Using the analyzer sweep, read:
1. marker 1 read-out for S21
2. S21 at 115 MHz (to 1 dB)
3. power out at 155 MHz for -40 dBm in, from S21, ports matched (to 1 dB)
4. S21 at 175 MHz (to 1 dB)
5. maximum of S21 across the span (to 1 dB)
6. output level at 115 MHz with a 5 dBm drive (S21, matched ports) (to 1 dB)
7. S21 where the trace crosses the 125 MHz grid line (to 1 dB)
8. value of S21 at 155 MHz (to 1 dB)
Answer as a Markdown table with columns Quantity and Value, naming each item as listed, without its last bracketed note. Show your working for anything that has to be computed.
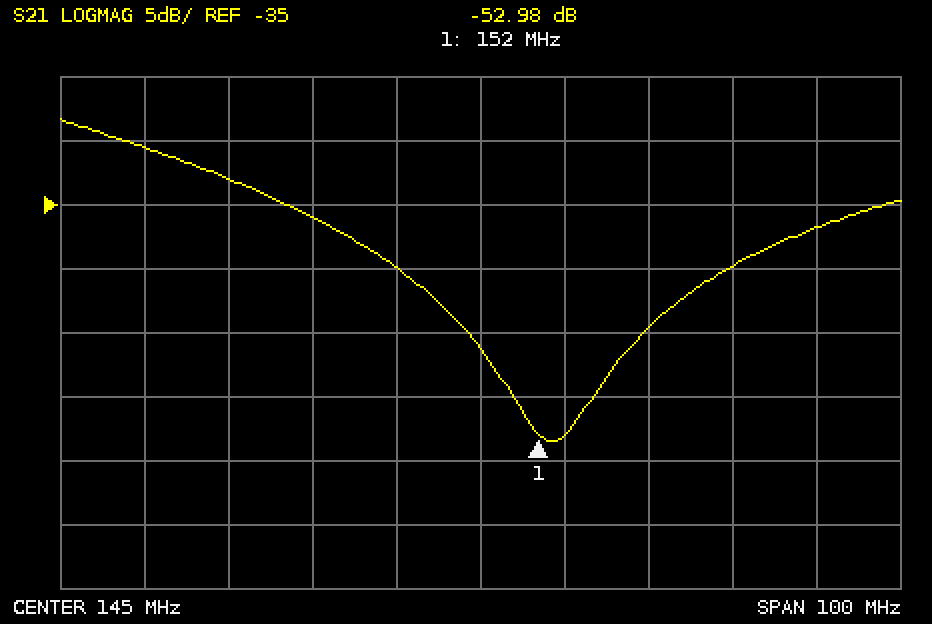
| Quantity | Value |
|---|---|
| marker 1 read-out for S21 | -52.98 dB |
| S21 at 115 MHz | -33 dB |
| power out at 155 MHz for -40 dBm in, from S21, ports matched | -40 dBm + (-53 dB) = -93 dBm |
| S21 at 175 MHz | -40 dB |
| maximum of S21 across the span | -28 dB |
| output level at 115 MHz with a 5 dBm drive (S21, matched ports) | 5 dBm + (-33 dB) = -28 dBm |
| S21 where the trace crosses the 125 MHz grid line | -36 dB |
| value of S21 at 155 MHz | -53 dB |
